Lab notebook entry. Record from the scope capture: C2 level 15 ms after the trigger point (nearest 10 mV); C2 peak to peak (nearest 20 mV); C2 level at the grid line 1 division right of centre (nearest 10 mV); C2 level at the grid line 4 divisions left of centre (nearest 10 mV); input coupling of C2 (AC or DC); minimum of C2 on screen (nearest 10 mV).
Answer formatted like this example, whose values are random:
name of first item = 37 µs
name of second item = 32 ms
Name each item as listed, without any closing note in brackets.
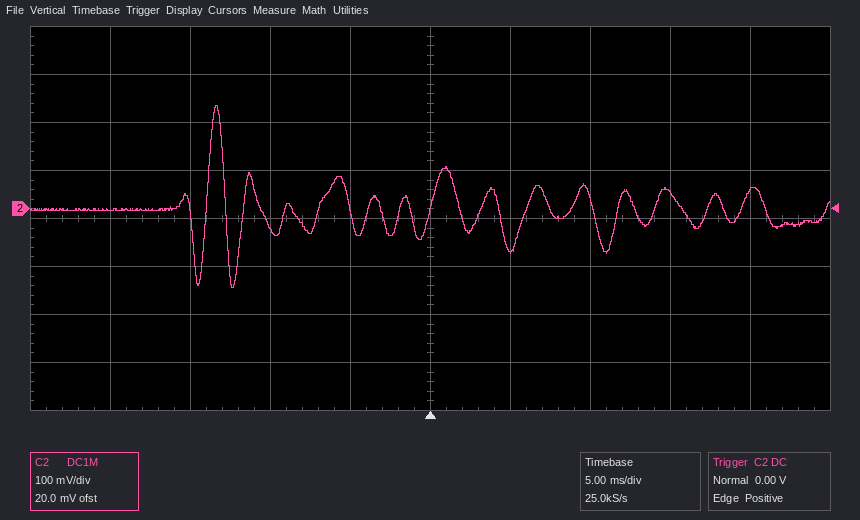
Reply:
C2 level 15 ms after the trigger point = 30 mV
C2 peak to peak = 380 mV
C2 level at the grid line 1 division right of centre = -80 mV
C2 level at the grid line 4 divisions left of centre = 0 mV
input coupling of C2 = DC
minimum of C2 on screen = -160 mV
